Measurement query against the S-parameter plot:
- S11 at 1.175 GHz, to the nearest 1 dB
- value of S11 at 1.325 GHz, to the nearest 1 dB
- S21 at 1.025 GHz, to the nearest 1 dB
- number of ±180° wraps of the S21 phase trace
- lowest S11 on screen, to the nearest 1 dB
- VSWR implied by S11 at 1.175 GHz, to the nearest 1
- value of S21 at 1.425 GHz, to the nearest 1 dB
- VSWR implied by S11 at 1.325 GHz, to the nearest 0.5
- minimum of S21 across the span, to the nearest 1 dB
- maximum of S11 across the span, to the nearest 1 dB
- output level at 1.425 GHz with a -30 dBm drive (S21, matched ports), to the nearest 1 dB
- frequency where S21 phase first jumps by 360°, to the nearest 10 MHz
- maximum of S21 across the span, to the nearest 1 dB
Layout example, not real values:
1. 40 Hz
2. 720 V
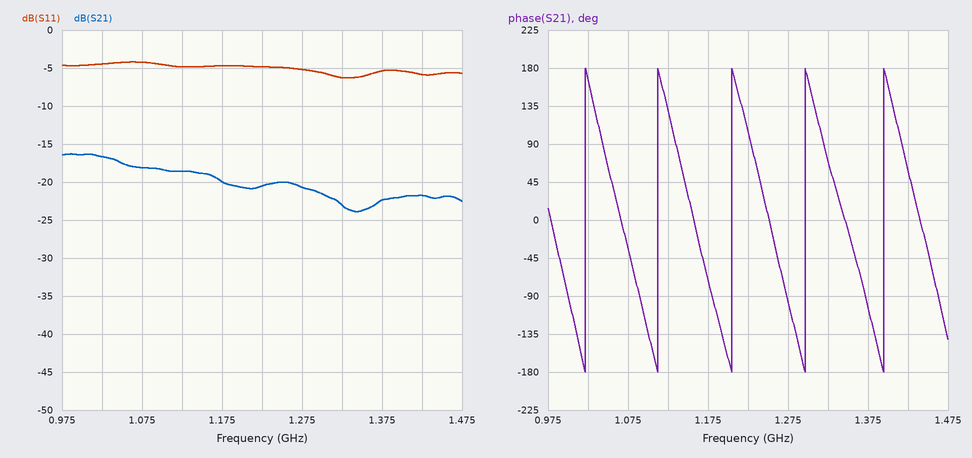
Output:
1. -5 dB
2. -6 dB
3. -17 dB
4. 5
5. -6 dB
6. 4
7. -22 dB
8. 3.0
9. -24 dB
10. -4 dB
11. -52 dBm
12. 1.02 GHz
13. -16 dB
